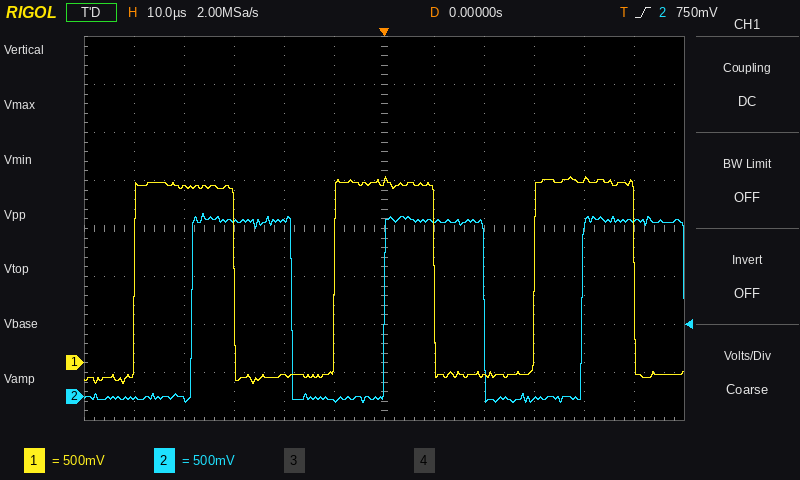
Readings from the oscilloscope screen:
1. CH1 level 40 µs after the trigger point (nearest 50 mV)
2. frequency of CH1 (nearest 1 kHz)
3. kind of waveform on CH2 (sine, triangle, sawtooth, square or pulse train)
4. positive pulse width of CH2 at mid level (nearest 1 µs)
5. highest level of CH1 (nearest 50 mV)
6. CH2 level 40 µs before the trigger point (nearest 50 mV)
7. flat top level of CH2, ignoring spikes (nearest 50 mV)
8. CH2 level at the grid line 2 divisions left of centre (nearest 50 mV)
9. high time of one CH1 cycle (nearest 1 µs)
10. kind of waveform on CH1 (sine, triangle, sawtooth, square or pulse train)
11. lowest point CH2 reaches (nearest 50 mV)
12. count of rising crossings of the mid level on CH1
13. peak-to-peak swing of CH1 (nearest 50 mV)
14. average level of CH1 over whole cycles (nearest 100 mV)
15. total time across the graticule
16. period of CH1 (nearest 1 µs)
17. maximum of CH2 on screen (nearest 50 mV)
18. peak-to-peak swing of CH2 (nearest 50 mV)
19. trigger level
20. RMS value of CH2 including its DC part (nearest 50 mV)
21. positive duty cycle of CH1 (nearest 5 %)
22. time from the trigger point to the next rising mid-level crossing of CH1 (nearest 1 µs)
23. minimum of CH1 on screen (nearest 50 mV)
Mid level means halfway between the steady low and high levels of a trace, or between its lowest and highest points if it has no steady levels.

1.90 V
25 kHz
square
20 µs
1.95 V
-50 mV
1.85 V
1.85 V
20 µs
square
-50 mV
3
2.15 V
900 mV
120 µs
40 µs
1.90 V
1.95 V
750 mV
1.30 V
50 %
30 µs
-200 mV
